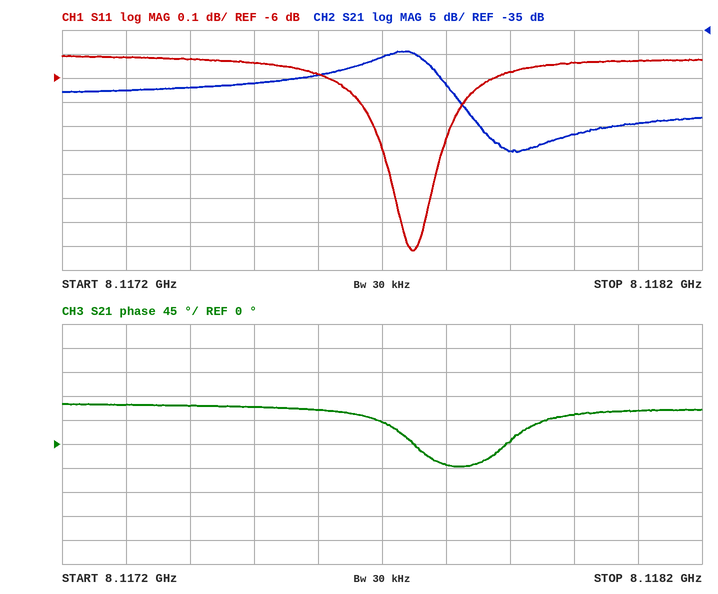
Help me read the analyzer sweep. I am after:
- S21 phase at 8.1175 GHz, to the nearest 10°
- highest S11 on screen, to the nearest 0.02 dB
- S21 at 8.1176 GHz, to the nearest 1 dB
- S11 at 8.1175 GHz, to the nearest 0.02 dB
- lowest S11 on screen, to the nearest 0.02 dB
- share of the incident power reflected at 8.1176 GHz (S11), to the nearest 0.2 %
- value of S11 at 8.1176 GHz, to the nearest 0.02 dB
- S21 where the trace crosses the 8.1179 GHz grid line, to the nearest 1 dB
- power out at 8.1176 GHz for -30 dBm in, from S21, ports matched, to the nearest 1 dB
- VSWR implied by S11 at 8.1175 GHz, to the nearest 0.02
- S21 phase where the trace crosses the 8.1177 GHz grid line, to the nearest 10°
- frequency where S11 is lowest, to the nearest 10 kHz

70°
-5.90 dB
-44 dB
-5.94 dB
-6.72 dB
25.2 %
-5.98 dB
-60 dB
-74 dBm
3.04
40°
8.11775 GHz
